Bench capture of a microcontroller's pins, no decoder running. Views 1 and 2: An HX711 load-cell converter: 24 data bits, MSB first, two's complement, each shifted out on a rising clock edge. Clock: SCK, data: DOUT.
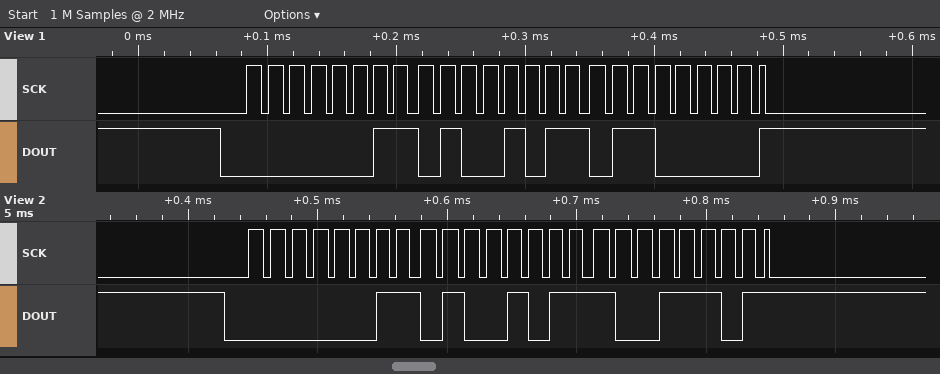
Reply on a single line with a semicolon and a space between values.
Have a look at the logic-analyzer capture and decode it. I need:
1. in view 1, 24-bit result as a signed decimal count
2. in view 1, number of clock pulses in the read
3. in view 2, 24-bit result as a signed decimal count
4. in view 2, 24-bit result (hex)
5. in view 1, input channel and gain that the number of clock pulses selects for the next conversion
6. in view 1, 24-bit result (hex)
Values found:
215904; 25; 215965; 0x034B9D; channel A, gain 128; 0x034B60
